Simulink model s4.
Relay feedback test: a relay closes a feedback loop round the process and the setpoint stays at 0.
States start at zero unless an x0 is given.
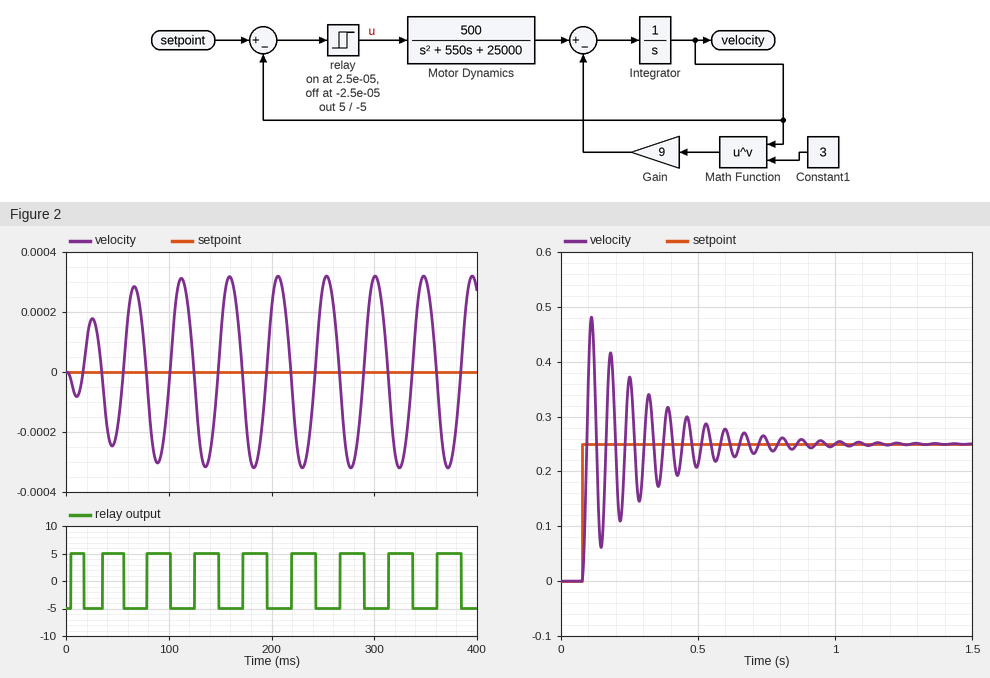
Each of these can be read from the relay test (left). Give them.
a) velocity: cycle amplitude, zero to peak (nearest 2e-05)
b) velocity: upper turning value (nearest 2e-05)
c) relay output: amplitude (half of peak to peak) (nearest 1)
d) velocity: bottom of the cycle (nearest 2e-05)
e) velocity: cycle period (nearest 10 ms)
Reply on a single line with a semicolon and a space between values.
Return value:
0.00032; 0.00032; 5; -0.00032; 50 ms
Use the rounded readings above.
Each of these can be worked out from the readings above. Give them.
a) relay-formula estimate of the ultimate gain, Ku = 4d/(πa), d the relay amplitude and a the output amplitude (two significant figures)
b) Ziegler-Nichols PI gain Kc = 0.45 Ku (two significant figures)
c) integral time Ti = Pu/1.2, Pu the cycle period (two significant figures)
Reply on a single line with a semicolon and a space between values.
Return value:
20000; 9000; 42 ms
